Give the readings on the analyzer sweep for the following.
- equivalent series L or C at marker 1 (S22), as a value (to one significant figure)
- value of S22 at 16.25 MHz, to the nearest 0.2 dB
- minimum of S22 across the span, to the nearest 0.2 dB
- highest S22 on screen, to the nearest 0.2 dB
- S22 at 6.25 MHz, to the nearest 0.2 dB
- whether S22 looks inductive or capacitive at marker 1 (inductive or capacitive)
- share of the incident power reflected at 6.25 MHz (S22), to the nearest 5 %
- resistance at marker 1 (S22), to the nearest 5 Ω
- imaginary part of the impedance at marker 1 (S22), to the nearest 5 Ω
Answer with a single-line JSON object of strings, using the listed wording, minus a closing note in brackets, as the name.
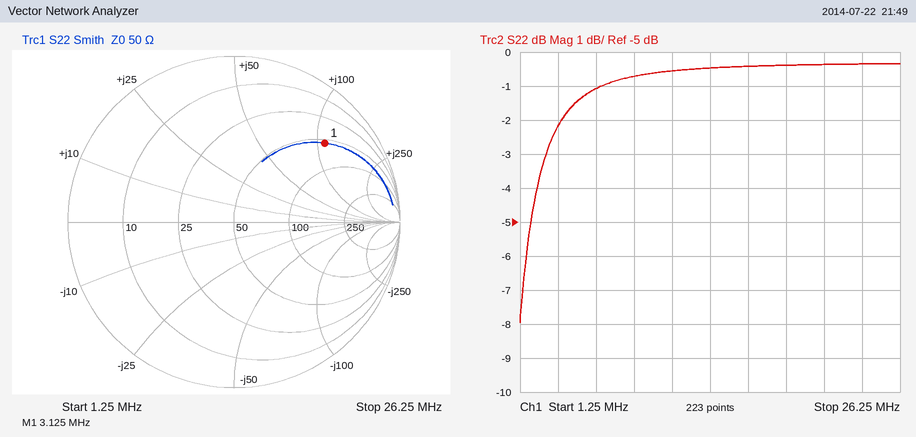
{"equivalent series L or C at marker 1 (S22), as a value": "6 µH", "value of S22 at 16.25 MHz, to the nearest 0.2 dB": "-0.4 dB", "minimum of S22 across the span, to the nearest 0.2 dB": "-8.0 dB", "highest S22 on screen, to the nearest 0.2 dB": "-0.4 dB", "S22 at 6.25 MHz, to the nearest 0.2 dB": "-1.0 dB", "whether S22 looks inductive or capacitive at marker 1": "inductive", "share of the incident power reflected at 6.25 MHz (S22), to the nearest 5 %": "80 %", "resistance at marker 1 (S22), to the nearest 5 Ω": "55 Ω", "imaginary part of the impedance at marker 1 (S22), to the nearest 5 Ω": "+110 Ω"}
